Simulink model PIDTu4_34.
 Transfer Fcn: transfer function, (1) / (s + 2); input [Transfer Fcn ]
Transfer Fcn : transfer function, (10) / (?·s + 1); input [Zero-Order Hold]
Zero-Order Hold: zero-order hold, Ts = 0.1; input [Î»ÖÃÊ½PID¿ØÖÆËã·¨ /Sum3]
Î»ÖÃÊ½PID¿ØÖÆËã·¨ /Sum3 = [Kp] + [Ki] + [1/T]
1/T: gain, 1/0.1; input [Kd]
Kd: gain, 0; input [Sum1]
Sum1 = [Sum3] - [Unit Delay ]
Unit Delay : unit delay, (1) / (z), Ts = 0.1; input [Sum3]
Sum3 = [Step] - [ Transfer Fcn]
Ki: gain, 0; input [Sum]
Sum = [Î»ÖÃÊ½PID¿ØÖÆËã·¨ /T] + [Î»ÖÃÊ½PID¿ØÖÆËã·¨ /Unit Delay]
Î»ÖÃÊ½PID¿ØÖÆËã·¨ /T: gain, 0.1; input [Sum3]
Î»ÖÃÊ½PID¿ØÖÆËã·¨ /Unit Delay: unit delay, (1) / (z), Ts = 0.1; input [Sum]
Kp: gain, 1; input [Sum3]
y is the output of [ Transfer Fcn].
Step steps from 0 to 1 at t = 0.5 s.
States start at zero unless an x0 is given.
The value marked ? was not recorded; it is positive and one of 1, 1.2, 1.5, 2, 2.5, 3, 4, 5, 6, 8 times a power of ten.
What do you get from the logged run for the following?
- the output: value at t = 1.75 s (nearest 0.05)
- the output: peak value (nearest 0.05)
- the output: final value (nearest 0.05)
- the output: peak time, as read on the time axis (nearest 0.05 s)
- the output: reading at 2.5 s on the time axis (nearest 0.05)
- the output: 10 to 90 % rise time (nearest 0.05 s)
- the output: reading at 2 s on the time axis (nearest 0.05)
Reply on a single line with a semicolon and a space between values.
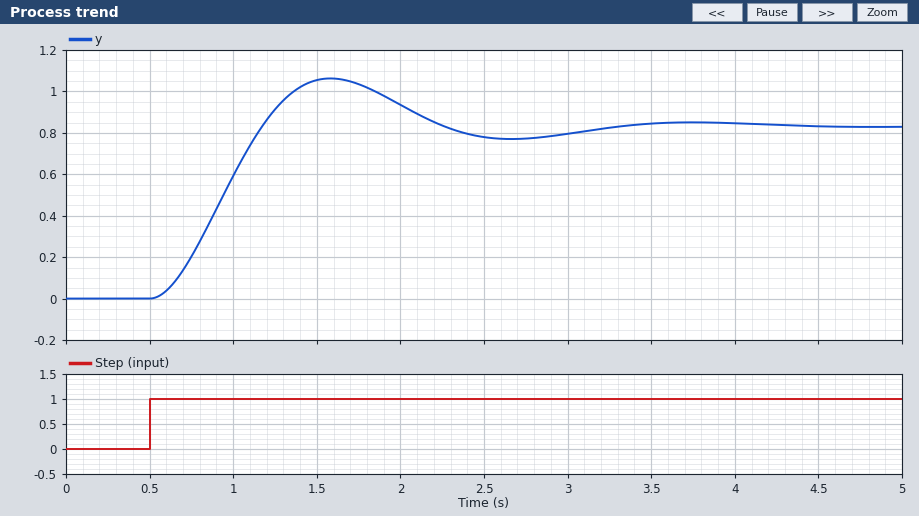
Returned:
1.05; 1.05; 0.85; 1.60 s; 0.80; 0.45 s; 0.95
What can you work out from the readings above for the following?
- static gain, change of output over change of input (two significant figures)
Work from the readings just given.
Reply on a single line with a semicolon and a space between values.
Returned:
0.85
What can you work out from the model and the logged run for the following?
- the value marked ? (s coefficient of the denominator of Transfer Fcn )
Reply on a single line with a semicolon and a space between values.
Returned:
1.2
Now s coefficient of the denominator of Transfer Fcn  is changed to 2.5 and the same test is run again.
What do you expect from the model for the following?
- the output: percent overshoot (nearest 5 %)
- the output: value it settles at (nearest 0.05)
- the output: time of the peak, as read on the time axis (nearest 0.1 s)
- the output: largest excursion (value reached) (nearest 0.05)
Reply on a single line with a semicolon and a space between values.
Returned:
15 %; 0.85; 2.2 s; 0.95
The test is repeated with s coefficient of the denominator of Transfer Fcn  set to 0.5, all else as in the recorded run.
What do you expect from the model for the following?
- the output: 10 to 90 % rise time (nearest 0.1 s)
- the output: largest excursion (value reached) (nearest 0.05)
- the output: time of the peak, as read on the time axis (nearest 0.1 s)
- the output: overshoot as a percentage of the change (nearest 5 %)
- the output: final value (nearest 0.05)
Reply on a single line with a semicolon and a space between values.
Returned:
0.3 s; 1.15; 1.2 s; 35 %; 0.85
